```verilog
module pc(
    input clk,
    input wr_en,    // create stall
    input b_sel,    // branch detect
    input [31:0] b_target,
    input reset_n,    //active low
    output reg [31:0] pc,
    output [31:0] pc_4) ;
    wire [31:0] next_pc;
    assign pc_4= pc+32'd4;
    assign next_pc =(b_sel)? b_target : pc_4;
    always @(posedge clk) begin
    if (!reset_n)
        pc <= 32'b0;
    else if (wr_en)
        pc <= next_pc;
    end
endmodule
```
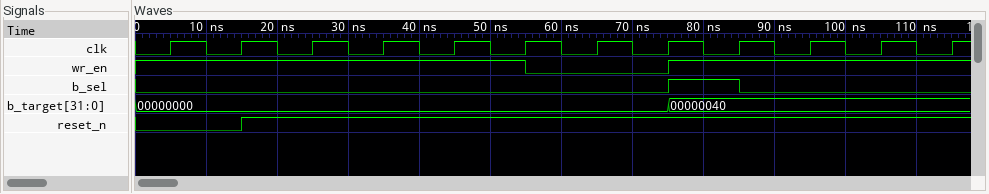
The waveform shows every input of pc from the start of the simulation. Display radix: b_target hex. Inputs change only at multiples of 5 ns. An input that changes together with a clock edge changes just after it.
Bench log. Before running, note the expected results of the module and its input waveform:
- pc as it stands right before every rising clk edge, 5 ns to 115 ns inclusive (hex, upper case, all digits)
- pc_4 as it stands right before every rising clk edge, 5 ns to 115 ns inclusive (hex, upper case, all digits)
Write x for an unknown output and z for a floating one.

x, 00000000, 00000000, 00000004, 00000008, 0000000C, 00000010, 00000010, 00000010, 00000040, 00000044, 00000048
x, 00000004, 00000004, 00000008, 0000000C, 00000010, 00000014, 00000014, 00000014, 00000044, 00000048, 0000004C
